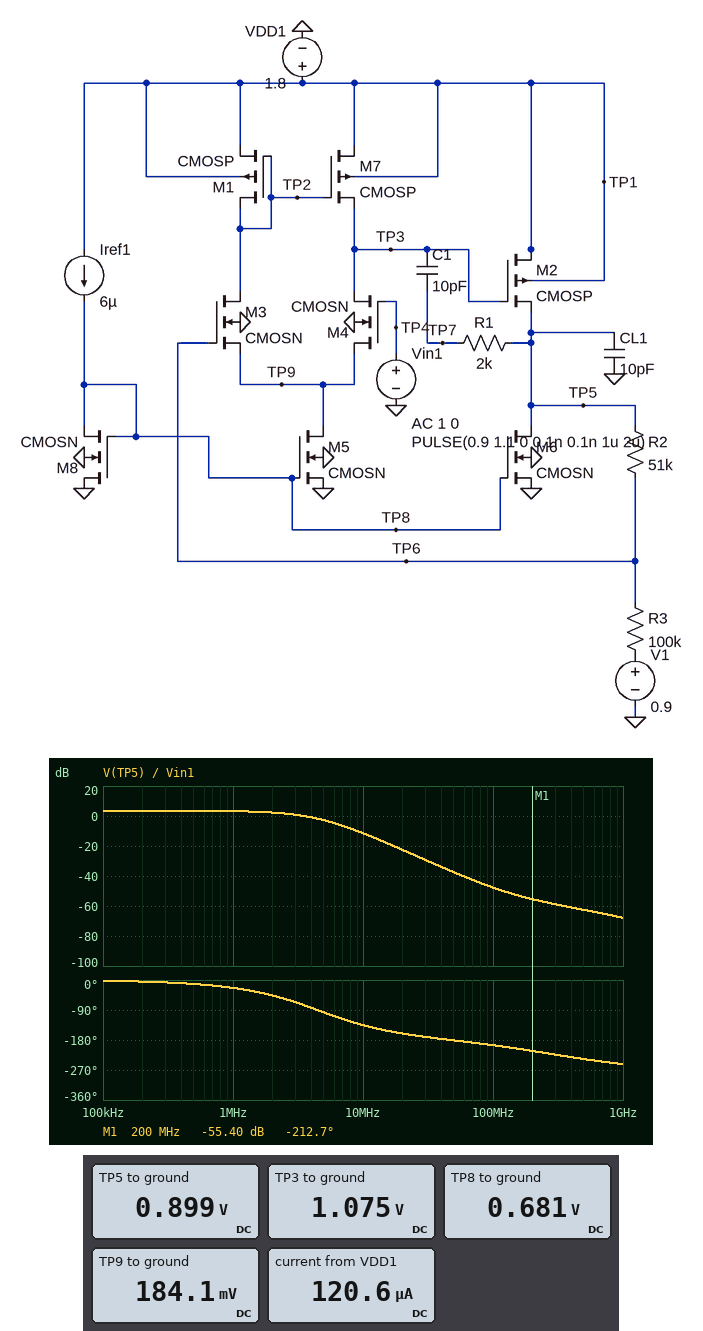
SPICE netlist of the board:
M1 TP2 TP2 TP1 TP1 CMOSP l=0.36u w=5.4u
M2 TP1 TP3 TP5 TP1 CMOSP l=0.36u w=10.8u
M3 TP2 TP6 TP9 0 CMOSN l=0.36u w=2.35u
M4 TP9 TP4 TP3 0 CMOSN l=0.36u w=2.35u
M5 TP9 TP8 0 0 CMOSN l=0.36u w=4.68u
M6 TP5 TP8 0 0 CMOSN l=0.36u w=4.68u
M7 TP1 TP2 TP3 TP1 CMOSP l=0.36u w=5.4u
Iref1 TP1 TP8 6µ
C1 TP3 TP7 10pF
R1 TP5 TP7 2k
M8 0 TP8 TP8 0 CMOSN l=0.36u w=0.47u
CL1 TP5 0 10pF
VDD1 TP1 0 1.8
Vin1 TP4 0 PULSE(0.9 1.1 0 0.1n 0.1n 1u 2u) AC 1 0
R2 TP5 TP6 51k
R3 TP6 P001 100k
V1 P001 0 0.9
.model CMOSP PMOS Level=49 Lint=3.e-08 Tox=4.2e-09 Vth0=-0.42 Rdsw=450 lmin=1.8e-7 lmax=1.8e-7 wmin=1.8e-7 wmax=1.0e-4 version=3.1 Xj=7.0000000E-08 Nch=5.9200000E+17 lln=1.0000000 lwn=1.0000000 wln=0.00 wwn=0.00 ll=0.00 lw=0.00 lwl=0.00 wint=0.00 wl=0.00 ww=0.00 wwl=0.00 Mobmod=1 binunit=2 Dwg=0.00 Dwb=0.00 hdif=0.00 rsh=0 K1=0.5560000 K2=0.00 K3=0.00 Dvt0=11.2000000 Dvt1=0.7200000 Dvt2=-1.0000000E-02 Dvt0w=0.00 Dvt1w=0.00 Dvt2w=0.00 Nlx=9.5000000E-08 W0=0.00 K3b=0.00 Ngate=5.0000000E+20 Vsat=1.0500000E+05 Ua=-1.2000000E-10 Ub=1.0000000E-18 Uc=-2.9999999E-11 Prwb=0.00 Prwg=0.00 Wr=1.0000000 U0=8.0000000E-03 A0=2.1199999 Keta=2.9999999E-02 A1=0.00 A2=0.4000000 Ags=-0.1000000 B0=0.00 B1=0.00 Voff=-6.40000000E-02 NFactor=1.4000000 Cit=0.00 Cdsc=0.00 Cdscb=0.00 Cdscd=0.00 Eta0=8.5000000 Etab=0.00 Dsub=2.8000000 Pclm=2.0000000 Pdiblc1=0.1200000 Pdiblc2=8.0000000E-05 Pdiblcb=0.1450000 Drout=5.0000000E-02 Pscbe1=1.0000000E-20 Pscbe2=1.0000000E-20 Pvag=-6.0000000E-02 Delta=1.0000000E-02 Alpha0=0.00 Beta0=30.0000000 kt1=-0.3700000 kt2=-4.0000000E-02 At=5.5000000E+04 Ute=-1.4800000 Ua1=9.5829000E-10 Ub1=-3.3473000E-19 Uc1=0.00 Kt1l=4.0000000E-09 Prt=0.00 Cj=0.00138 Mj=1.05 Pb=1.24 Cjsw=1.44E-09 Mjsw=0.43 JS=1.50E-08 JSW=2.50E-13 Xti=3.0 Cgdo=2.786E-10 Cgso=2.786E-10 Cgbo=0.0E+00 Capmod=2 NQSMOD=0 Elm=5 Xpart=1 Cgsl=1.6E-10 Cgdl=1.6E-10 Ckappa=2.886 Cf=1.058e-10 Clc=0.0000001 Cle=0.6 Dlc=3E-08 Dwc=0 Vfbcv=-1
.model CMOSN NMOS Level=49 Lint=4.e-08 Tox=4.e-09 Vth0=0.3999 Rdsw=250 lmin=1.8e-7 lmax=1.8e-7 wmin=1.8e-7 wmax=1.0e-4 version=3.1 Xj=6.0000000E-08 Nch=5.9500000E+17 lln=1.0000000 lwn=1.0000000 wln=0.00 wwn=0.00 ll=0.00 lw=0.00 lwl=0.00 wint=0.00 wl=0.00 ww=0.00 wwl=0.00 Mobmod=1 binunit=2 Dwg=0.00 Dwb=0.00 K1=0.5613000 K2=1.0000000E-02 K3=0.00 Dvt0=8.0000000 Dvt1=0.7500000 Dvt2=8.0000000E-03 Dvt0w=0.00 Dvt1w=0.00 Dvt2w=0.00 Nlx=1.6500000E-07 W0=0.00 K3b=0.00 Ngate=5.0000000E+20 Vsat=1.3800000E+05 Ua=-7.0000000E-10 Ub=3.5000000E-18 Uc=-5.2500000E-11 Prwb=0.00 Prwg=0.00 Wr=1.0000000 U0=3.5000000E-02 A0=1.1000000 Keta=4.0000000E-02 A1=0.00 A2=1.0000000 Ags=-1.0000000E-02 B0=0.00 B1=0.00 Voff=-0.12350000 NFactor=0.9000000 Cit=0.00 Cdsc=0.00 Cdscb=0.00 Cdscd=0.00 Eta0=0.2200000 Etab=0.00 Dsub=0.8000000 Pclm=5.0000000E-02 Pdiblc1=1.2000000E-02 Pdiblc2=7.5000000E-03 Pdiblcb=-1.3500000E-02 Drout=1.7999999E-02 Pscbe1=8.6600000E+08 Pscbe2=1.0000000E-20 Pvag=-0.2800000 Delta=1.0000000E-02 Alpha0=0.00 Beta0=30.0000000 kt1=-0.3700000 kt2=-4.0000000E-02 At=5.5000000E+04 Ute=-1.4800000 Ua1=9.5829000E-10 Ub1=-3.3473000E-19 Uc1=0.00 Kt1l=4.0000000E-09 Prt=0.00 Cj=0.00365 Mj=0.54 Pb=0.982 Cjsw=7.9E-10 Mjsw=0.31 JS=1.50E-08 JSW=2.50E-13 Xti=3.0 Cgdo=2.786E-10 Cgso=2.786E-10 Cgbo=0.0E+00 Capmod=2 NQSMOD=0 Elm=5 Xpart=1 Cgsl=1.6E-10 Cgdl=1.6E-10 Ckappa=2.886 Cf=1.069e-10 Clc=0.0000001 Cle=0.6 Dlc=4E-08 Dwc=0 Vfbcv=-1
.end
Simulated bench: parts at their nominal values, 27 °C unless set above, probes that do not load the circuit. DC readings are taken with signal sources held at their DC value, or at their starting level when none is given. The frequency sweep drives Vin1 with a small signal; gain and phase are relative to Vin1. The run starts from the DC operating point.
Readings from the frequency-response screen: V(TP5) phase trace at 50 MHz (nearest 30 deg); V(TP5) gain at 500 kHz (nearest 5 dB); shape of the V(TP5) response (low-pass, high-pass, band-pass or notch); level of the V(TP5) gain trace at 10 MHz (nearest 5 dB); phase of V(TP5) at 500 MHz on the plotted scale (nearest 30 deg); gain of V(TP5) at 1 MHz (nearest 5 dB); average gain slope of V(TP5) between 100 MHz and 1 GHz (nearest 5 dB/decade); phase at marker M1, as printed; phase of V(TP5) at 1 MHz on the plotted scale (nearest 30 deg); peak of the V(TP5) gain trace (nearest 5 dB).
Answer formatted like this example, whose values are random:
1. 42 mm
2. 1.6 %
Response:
1. -180 deg
2. 5 dB
3. low-pass
4. -10 dB
5. -240 deg
6. 5 dB
7. -20 dB/decade
8. -212.7 deg
9. -30 deg
10. 5 dB
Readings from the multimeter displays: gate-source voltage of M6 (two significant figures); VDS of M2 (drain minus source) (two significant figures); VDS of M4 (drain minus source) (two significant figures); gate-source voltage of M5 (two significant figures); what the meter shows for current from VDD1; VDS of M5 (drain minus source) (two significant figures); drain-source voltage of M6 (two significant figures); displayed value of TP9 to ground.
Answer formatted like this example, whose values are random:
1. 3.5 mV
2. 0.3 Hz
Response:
1. 680 mV
2. 900 mV
3. -890 mV
4. 680 mV
5. 120.6 µA
6. 180 mV
7. 900 mV
8. 184.1 mV
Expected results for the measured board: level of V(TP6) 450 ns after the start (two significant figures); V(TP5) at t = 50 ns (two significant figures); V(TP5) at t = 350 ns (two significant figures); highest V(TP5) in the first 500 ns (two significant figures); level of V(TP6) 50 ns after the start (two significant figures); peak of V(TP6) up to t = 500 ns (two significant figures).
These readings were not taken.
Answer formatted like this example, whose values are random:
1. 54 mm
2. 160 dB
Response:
1. 1.1 V
2. 1.0 V
3. 1.2 V
4. 1.2 V
5. 980 mV
6. 1.1 V
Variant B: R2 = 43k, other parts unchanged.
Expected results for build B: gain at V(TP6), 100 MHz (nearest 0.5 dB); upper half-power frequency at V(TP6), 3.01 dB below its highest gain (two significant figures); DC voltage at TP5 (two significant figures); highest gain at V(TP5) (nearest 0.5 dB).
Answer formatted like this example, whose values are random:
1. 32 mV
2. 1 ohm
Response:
1. -26.0 dB
2. 3.4 MHz
3. 900 mV
4. 3.0 dB
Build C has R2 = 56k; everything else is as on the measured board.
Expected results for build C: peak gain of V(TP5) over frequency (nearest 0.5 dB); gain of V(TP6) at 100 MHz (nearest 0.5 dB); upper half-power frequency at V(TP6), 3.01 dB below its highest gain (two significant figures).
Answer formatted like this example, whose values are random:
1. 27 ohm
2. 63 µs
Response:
1. 4.0 dB
2. -24.5 dB
3. 3.1 MHz
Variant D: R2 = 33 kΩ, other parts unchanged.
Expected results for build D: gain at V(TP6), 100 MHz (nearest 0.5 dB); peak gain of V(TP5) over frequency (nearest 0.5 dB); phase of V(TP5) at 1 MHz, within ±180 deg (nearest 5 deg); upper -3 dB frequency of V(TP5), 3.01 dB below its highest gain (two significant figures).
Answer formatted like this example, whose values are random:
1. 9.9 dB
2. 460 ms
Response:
1. -27.5 dB
2. 2.5 dB
3. -20 deg
4. 3.7 MHz
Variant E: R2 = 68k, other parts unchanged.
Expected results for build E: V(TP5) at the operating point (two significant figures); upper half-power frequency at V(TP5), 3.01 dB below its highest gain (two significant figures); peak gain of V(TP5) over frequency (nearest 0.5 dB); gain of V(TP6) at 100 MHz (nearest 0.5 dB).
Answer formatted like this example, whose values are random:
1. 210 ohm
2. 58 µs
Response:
1. 900 mV
2. 2.8 MHz
3. 4.5 dB
4. -23.5 dB
